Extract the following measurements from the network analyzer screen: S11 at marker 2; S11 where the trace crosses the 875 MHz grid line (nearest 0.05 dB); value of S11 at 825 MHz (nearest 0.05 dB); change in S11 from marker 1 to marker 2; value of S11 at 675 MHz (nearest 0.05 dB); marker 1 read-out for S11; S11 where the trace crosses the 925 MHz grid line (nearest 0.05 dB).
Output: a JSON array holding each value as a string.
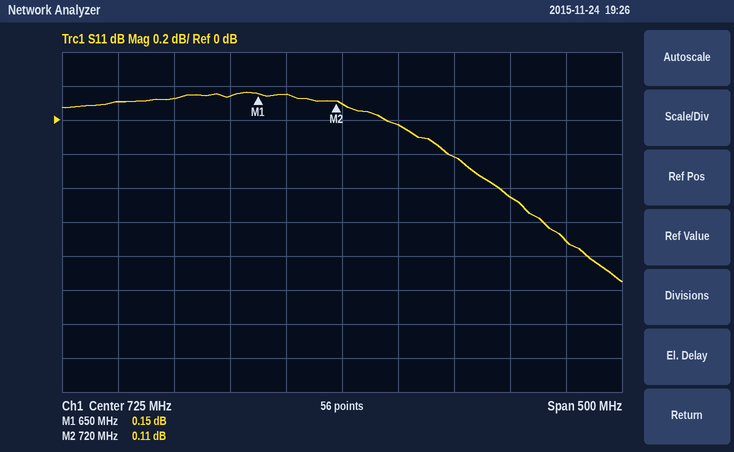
["0.11 dB", "-0.45 dB", "-0.20 dB", "-0.04 dB", "0.15 dB", "0.15 dB", "-0.70 dB"]
